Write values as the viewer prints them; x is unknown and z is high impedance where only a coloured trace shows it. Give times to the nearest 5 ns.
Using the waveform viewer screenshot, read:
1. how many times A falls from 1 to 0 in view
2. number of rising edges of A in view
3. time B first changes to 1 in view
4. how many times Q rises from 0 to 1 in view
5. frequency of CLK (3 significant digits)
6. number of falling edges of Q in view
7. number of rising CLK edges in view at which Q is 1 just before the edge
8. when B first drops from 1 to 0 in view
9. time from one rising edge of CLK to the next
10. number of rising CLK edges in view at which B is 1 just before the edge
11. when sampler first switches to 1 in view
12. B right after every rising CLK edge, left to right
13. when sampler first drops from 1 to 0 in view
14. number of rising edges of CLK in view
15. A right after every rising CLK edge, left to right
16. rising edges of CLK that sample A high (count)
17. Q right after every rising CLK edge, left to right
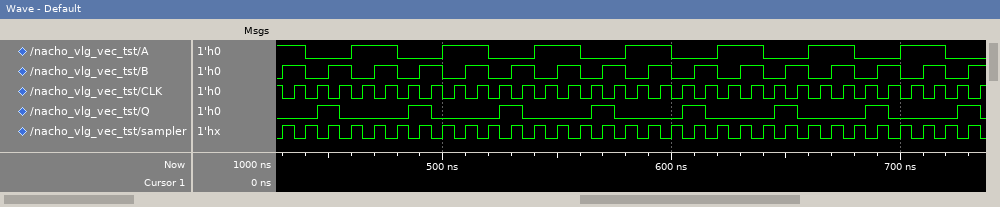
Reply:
8
7
430 ns
8
100 MHz
8
8
440 ns
10 ns
16
430 ns
1 0 1 0 1 0 1 0 1 0 1 0 1 0 1 0 1 0 1 0 1 0 1 0 1 0 1 0 1 0 1
435 ns
31
1 0 0 1 1 0 0 1 1 0 0 1 1 0 0 1 1 0 0 1 1 0 0 1 1 0 0 1 1 0 0
15
0 1 0 0 0 1 0 0 0 1 0 0 0 1 0 0 0 1 0 0 0 1 0 0 0 1 0 0 0 1 0
